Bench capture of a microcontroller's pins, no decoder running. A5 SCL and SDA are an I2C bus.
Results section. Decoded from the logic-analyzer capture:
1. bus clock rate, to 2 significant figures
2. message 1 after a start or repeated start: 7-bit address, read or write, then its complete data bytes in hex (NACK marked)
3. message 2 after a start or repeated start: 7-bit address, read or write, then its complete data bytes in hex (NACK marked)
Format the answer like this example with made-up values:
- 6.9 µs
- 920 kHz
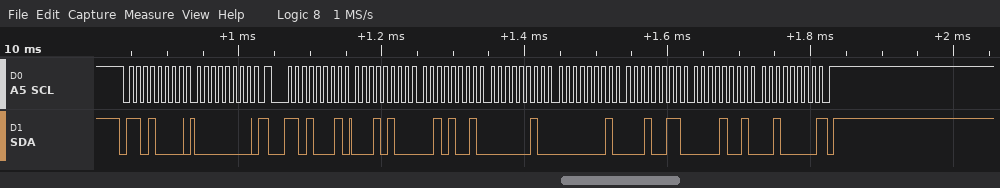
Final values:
- 100 kHz
- 0x68 write: 00
- 0x68 read: 14 29 02 01 13 09 20 NACK
